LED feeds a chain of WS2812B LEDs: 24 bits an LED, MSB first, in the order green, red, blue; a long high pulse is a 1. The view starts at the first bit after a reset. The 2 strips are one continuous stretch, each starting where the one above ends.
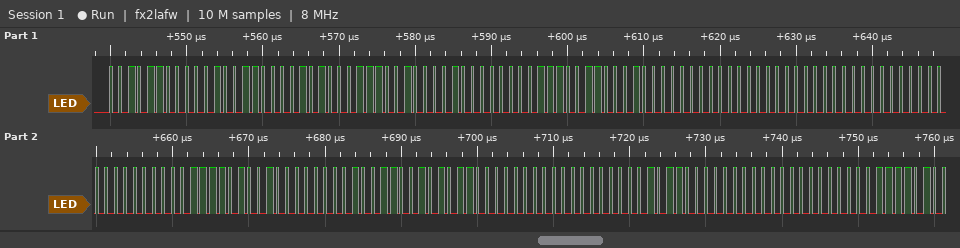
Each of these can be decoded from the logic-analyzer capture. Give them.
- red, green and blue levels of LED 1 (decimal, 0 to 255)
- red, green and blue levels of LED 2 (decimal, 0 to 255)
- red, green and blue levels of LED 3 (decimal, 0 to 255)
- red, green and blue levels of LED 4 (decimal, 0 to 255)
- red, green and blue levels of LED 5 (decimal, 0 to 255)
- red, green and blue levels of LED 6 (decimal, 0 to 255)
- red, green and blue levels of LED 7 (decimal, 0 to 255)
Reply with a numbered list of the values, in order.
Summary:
1. 19, 44, 10
2. 8, 57, 7
3. 0, 49, 0
4. 0, 0, 0
5. 32, 61, 19
6. 0, 43, 0
7. 0, 44, 0
